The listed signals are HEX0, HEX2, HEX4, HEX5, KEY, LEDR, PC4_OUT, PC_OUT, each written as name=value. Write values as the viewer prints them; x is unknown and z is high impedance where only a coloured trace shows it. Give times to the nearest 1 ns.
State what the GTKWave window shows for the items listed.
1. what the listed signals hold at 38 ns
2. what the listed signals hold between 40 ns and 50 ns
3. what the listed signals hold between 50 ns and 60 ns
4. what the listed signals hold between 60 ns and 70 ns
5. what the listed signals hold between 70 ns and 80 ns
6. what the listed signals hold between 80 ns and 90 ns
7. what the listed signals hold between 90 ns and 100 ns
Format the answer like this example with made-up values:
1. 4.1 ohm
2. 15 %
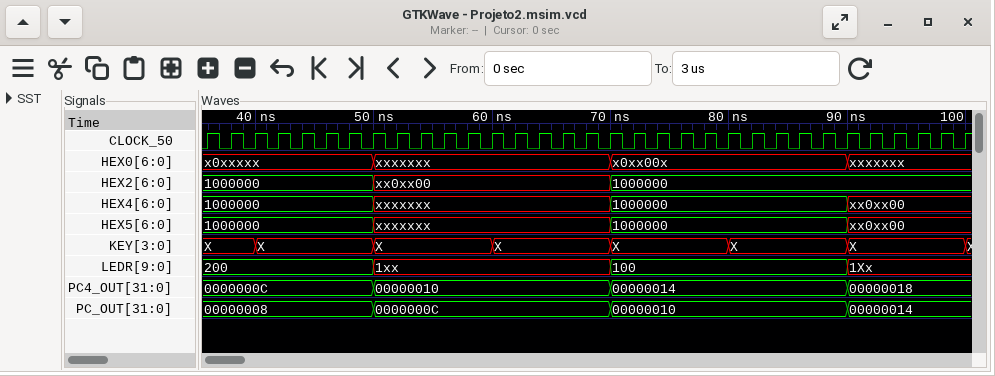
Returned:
1. HEX0=x0xxxxx, HEX2=1000000, HEX4=1000000, HEX5=1000000, KEY=X, LEDR=200, PC4_OUT=0000000C, PC_OUT=00000008
2. HEX0=x0xxxxx, HEX2=1000000, HEX4=1000000, HEX5=1000000, KEY=X, LEDR=200, PC4_OUT=0000000C, PC_OUT=00000008
3. HEX0=xxxxxxx, HEX2=xx0xx00, HEX4=xxxxxxx, HEX5=xxxxxxx, KEY=X, LEDR=1xx, PC4_OUT=00000010, PC_OUT=0000000C
4. HEX0=xxxxxxx, HEX2=xx0xx00, HEX4=xxxxxxx, HEX5=xxxxxxx, KEY=X, LEDR=1xx, PC4_OUT=00000010, PC_OUT=0000000C
5. HEX0=x0xx00x, HEX2=1000000, HEX4=1000000, HEX5=1000000, KEY=X, LEDR=100, PC4_OUT=00000014, PC_OUT=00000010
6. HEX0=x0xx00x, HEX2=1000000, HEX4=1000000, HEX5=1000000, KEY=X, LEDR=100, PC4_OUT=00000014, PC_OUT=00000010
7. HEX0=xxxxxxx, HEX2=1000000, HEX4=xx0xx00, HEX5=xx0xx00, KEY=X, LEDR=1Xx, PC4_OUT=00000018, PC_OUT=00000014
